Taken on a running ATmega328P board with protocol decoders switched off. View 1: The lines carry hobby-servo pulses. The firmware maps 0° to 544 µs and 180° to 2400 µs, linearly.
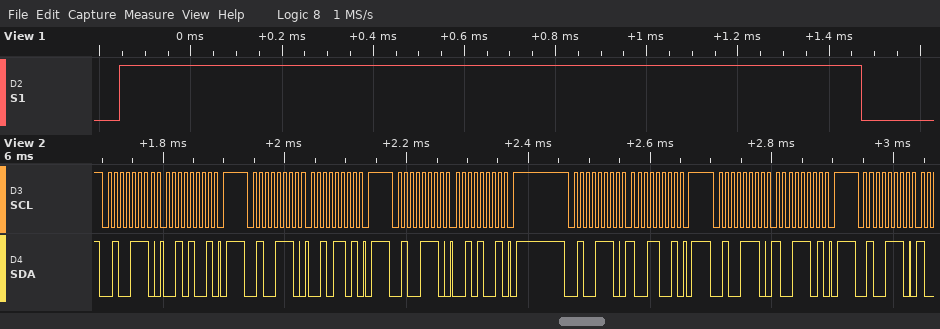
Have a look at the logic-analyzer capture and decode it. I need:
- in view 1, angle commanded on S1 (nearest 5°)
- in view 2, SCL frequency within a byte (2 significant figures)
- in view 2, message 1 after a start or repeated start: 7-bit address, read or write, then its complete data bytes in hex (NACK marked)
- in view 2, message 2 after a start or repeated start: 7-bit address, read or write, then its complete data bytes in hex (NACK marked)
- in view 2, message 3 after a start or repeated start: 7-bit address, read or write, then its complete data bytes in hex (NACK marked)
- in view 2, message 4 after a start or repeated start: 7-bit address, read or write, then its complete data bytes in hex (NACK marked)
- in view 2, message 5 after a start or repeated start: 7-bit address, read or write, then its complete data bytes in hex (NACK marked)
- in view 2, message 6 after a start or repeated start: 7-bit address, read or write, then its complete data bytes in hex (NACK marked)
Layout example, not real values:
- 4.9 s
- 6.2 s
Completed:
- 105°
- 100 kHz
- 0x27 write: 29
- 0x27 write: 2D
- 0x27 write: 29
- 0x27 write: 99
- 0x27 write: 9D
- 0x27 write
